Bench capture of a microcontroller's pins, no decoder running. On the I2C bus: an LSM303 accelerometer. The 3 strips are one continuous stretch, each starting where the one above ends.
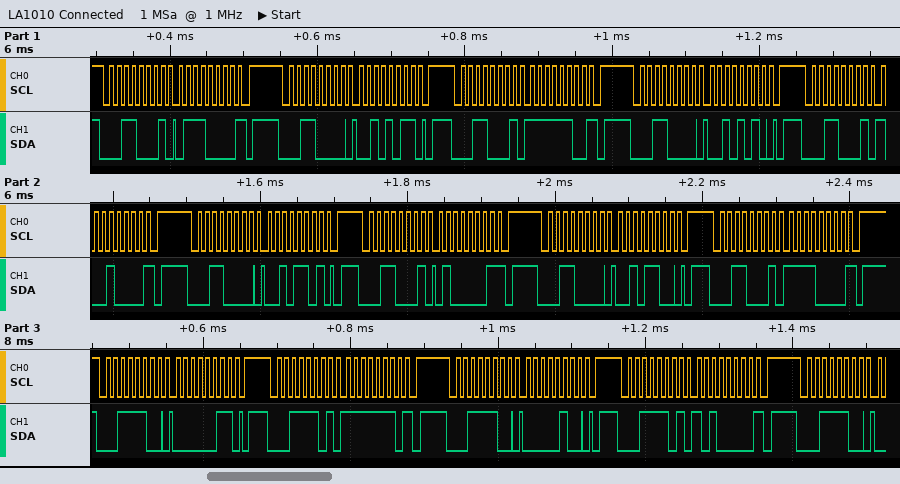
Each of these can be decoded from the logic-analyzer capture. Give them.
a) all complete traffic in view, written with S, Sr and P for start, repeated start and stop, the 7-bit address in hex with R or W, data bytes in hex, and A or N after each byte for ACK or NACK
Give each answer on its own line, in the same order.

S 18R A 70 N P S 18W A 2B A P S 18R A FC N P S 18W A 2A A P S 18R A 90 N P S 18W A 2D A P S 18R A 41 N P S 18W A 2C A P S 18R A F0 N P S 1EW A 03 A P S 1ER A FE N P S 1EW A 04 A P S 1ER A A0 N P S 1EW A
